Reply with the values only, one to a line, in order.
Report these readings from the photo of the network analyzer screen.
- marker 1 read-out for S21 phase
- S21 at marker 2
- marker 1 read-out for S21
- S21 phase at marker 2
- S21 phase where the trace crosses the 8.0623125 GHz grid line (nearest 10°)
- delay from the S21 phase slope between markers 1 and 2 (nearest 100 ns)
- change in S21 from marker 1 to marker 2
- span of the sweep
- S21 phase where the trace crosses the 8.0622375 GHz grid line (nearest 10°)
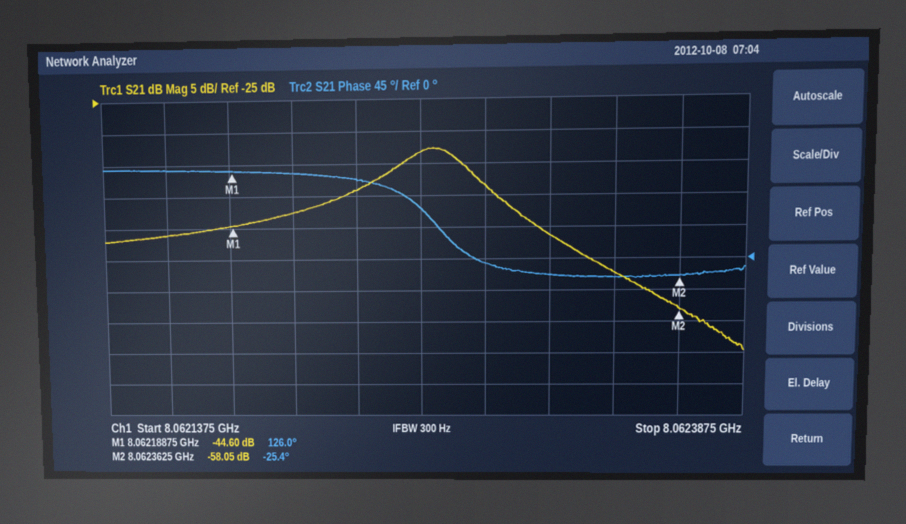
126.0°
-58.05 dB
-44.60 dB
-25.4°
-20°
2.4 µs
-13.45 dB
250 kHz
110°
